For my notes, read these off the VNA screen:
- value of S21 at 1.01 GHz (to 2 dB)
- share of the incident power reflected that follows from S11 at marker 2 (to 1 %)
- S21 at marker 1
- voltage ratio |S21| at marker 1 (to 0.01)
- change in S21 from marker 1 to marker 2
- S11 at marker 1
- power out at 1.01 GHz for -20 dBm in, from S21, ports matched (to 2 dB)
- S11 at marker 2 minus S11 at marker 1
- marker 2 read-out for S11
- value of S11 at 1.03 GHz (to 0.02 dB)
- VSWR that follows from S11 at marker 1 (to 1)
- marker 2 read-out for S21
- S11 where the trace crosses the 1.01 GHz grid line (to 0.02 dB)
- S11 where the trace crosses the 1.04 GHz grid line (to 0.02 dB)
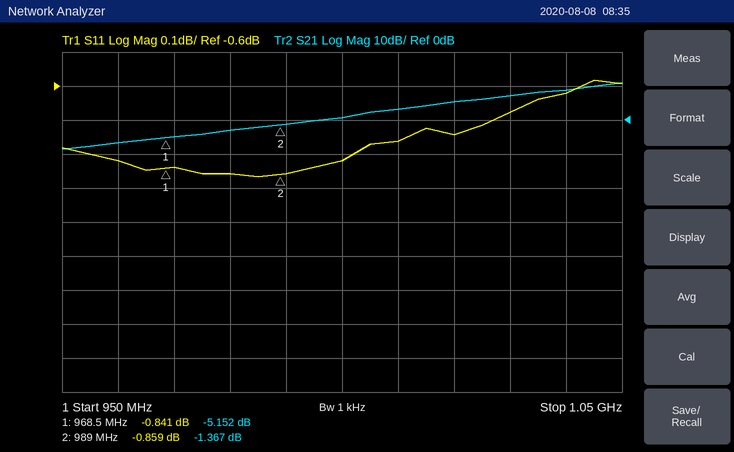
4 dB
82 %
-5.152 dB
0.55
3.785 dB
-0.841 dB
-16 dBm
-0.018 dB
-0.859 dB
-0.68 dB
21
-1.367 dB
-0.76 dB
-0.62 dB
